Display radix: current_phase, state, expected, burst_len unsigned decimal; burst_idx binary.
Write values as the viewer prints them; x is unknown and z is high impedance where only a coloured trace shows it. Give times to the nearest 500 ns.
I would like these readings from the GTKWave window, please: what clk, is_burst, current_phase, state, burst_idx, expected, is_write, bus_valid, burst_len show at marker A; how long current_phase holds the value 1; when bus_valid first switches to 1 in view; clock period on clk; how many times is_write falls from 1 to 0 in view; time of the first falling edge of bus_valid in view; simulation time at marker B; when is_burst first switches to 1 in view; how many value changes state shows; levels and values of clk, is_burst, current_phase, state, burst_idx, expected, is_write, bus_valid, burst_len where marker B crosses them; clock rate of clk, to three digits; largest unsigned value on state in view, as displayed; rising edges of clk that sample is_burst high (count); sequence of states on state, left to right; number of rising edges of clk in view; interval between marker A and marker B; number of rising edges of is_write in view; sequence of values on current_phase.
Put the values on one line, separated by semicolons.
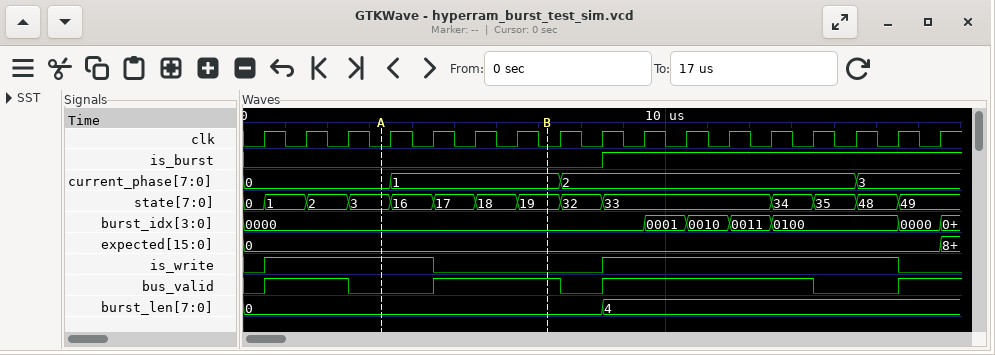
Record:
clk=0, is_burst=0, current_phase=0, state=3, burst_idx=0000, expected=0, is_write=1, bus_valid=0, burst_len=0; 4000 ns; 500 ns; 1000 ns; 2; 2500 ns; 7000 ns; 8500 ns; 13; clk=0, is_burst=0, current_phase=1, state=19, burst_idx=0000, expected=0, is_write=0, bus_valid=1, burst_len=0; 1.00 MHz; 49; 8; 0, 1, 2, 3, 16, 17, 18, 19, 32, 33, 34, 35, 48, 49; 17; 4000 ns; 2; 0, 1, 2, 3
